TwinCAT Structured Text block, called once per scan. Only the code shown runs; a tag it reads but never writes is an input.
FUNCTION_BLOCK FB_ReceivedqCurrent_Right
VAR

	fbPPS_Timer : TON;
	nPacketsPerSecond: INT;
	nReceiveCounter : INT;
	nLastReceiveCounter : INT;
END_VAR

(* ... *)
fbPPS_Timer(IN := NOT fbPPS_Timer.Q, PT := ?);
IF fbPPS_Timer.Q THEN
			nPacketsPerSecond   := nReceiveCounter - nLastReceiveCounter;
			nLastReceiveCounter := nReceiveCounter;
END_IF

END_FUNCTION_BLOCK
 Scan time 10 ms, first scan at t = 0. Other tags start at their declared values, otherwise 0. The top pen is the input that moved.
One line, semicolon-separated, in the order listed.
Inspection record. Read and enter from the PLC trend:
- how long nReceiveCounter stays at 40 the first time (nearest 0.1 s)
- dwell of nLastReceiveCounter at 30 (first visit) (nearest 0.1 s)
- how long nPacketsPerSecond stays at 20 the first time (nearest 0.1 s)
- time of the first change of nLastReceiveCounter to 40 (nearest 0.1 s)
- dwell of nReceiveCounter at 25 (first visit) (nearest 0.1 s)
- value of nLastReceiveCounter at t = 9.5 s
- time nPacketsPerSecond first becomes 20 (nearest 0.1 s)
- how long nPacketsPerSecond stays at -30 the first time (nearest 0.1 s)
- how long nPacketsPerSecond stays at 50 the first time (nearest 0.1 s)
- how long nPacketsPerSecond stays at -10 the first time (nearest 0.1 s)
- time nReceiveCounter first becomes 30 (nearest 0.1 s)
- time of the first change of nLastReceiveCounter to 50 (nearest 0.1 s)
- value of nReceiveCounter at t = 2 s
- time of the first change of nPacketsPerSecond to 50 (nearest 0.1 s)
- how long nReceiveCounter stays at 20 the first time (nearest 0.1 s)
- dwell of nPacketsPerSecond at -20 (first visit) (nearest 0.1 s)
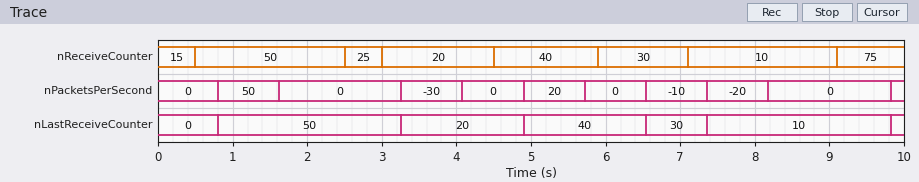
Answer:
1.4 s; 0.8 s; 0.8 s; 4.9 s; 0.5 s; 10; 4.9 s; 0.8 s; 0.8 s; 0.8 s; 5.9 s; 0.8 s; 50; 0.8 s; 1.5 s; 0.8 s
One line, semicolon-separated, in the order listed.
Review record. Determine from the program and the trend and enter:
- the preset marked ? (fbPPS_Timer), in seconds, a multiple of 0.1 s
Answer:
0.8 s
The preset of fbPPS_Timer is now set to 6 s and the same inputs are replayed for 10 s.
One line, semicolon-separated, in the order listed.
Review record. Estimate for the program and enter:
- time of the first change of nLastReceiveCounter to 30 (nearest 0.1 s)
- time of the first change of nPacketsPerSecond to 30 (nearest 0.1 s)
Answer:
6.0 s; 6.0 s
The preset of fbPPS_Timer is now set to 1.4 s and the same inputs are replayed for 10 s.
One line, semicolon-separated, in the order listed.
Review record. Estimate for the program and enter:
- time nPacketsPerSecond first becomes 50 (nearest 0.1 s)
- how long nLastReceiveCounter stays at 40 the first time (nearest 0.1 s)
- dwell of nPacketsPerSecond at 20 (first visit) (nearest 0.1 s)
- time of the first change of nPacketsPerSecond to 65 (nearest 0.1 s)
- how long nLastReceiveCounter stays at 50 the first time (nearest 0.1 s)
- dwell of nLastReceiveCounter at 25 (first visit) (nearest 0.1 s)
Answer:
1.4 s; 1.4 s; 1.4 s; 9.9 s; 1.4 s; 1.4 s
